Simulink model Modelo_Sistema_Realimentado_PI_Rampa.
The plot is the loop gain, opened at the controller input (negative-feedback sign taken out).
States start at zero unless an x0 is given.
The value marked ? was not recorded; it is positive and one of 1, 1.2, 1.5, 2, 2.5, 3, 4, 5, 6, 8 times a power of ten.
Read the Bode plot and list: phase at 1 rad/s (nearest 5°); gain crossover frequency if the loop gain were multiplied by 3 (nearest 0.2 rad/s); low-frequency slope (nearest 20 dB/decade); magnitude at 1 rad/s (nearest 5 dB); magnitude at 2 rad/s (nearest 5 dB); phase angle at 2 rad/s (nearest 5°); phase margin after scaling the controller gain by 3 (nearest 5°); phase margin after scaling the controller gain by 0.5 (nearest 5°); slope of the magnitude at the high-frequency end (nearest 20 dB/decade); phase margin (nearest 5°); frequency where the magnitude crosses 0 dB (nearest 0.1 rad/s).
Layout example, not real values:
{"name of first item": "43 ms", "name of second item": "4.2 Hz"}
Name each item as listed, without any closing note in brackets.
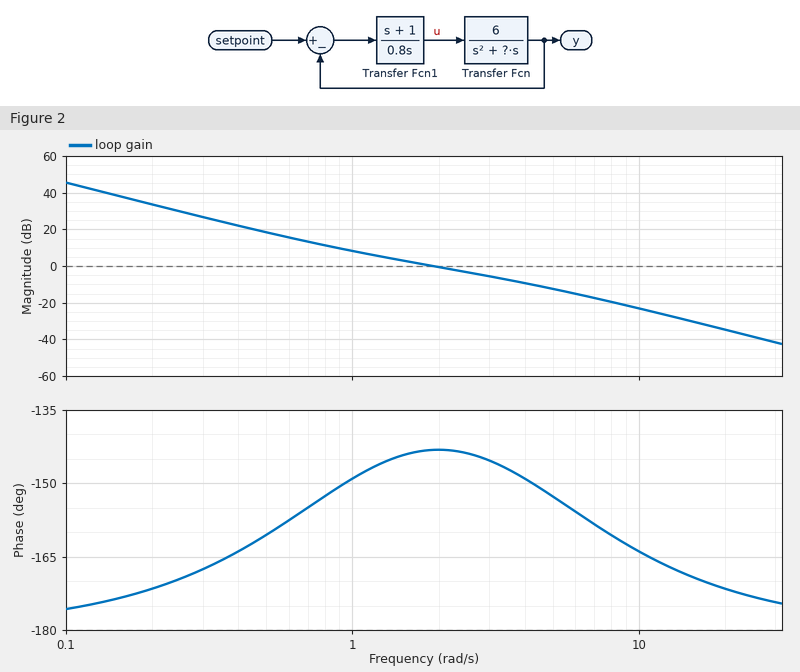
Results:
{"phase at 1 rad/s": "-150°", "gain crossover frequency if the loop gain were multiplied by 3": "4.0 rad/s", "low-frequency slope": "-40 dB/decade", "magnitude at 1 rad/s": "10 dB", "magnitude at 2 rad/s": "0 dB", "phase angle at 2 rad/s": "-145°", "phase margin after scaling the controller gain by 3": "30°", "phase margin after scaling the controller gain by 0.5": "35°", "slope of the magnitude at the high-frequency end": "-40 dB/decade", "phase margin": "35°", "frequency where the magnitude crosses 0 dB": "1.9 rad/s"}
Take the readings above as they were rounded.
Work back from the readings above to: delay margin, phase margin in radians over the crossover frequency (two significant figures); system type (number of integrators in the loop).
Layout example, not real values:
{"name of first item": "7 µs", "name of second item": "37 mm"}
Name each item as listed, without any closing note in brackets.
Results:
{"delay margin, phase margin in radians over the crossover frequency": "0.32 s", "system type": "2"}
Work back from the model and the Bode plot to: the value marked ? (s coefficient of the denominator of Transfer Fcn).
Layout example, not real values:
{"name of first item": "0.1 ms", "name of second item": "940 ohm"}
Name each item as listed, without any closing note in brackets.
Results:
{"the value marked ?": "4"}
